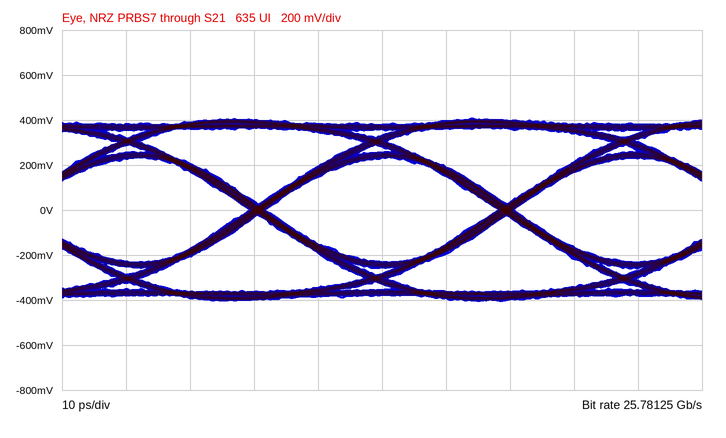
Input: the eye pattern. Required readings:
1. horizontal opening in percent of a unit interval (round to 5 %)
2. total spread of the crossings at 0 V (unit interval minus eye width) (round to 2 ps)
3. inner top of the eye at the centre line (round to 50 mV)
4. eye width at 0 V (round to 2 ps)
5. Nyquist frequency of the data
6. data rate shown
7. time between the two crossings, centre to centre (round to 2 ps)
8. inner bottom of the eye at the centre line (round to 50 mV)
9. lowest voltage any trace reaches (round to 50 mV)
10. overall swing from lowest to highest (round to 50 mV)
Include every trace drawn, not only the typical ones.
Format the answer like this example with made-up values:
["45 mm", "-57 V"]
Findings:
["95 %", "2 ps", "250 mV", "36 ps", "12.89062 GHz", "25.78125 Gb/s", "38 ps", "-250 mV", "-400 mV", "800 mV"]
